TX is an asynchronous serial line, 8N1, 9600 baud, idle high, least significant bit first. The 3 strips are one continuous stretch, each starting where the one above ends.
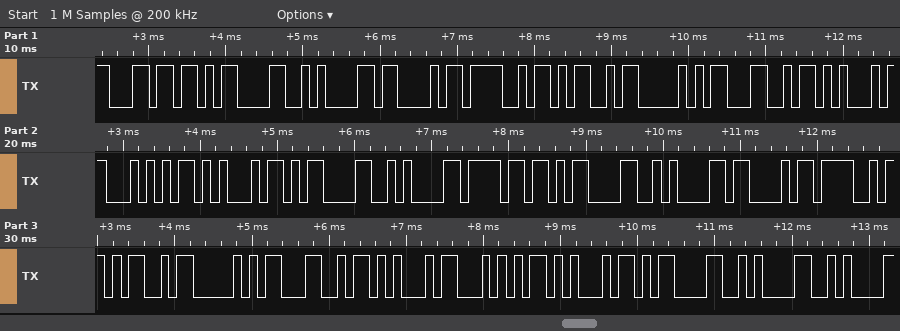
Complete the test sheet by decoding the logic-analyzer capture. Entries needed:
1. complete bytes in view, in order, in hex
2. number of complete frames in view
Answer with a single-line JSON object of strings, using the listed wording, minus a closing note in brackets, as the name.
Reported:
{"complete bytes in view, in order, in hex": "0x6C 0x0D 0x0A 0x43 0x4F 0x4D 0x50 0x4C 0x45 0x54 0x45 0x0D 0x0A 0x6F 0x0D 0x0A 0x43 0x4F 0x4D 0x50 0x4C 0x45 0x54 0x45 0x0D 0x0A 0x0A", "number of complete frames in view": "27"}
